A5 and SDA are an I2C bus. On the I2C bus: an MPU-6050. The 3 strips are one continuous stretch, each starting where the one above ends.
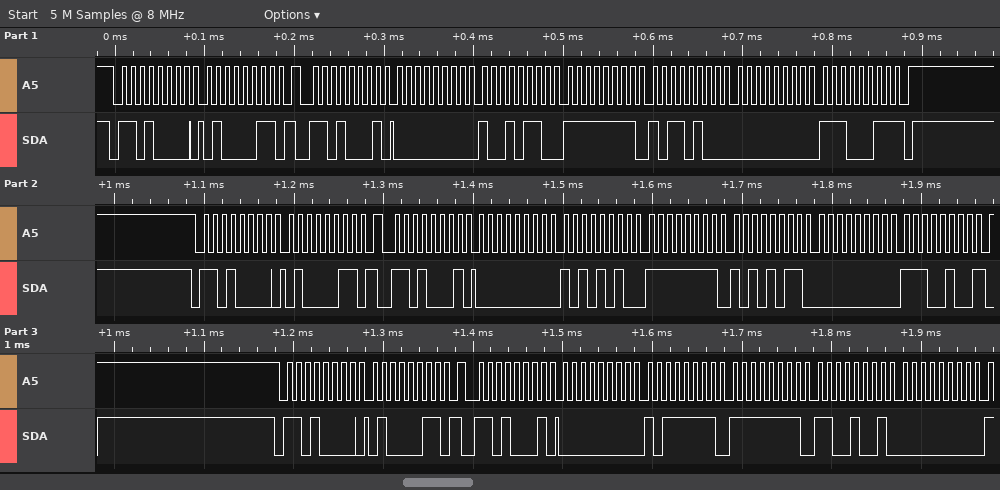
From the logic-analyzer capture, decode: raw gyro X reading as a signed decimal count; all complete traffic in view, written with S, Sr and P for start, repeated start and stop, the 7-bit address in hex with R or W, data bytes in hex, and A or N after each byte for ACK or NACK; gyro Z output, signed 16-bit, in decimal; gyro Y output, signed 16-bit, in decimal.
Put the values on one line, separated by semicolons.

150; S 68W A 43 A Sr 68R A 00 A 96 A FF A B4 A 00 A E3 N P S 68W A 43 A Sr 68R A 00 A AA A FF A AB A 00 A E4 N P S 68W A 43 A Sr 68R A 00 A BF A FF A C9 A 00 A; 227; -76
